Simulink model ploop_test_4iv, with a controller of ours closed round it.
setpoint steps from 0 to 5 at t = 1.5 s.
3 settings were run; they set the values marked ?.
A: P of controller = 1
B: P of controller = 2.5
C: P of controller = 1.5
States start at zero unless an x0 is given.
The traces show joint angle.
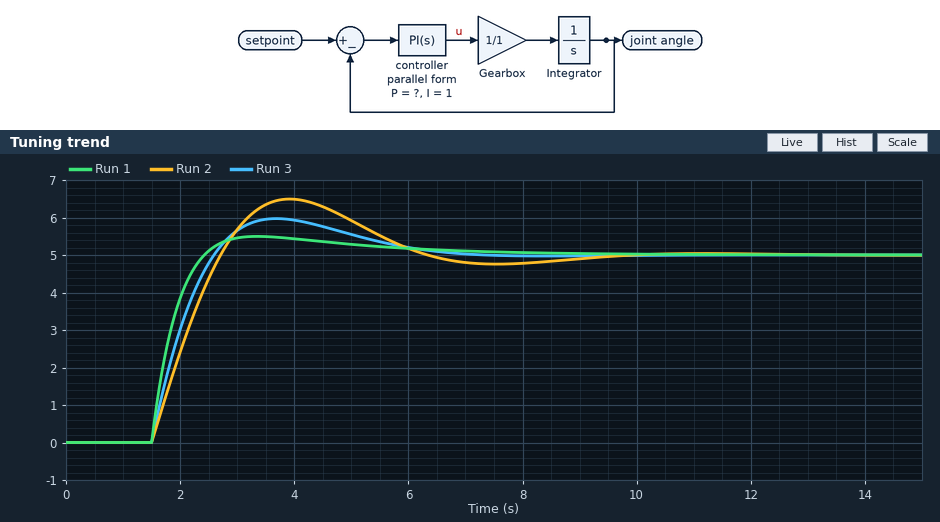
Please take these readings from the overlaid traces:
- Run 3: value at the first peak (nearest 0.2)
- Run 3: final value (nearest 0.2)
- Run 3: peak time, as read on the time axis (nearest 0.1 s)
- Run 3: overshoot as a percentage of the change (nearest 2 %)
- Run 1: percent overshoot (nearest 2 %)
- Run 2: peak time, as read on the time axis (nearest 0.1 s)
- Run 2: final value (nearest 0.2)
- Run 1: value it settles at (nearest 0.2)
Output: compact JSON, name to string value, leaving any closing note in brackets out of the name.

{"Run 3: value at the first peak": "6.0", "Run 3: final value": "5.0", "Run 3: peak time, as read on the time axis": "3.7 s", "Run 3: overshoot as a percentage of the change": "20 %", "Run 1: percent overshoot": "10 %", "Run 2: peak time, as read on the time axis": "3.9 s", "Run 2: final value": "5.0", "Run 1: value it settles at": "5.0"}
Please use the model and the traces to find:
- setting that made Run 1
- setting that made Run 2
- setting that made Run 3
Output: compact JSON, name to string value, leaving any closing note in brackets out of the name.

{"setting that made Run 1": "B", "setting that made Run 2": "A", "setting that made Run 3": "C"}
